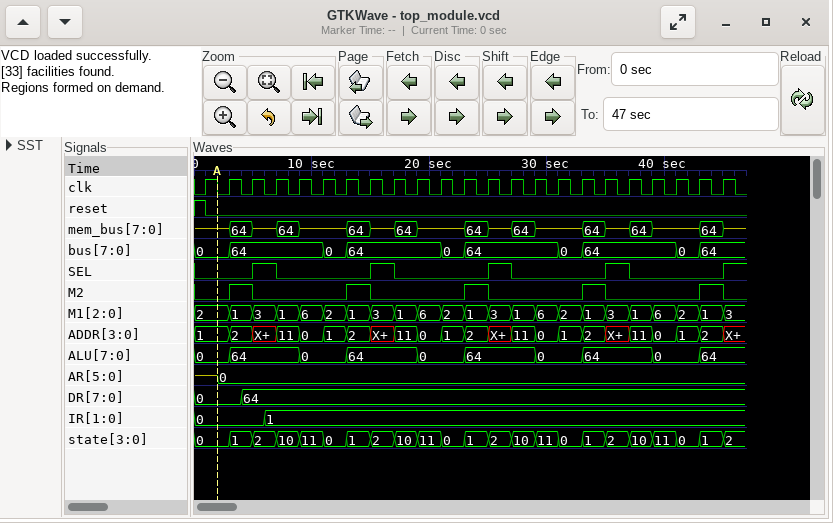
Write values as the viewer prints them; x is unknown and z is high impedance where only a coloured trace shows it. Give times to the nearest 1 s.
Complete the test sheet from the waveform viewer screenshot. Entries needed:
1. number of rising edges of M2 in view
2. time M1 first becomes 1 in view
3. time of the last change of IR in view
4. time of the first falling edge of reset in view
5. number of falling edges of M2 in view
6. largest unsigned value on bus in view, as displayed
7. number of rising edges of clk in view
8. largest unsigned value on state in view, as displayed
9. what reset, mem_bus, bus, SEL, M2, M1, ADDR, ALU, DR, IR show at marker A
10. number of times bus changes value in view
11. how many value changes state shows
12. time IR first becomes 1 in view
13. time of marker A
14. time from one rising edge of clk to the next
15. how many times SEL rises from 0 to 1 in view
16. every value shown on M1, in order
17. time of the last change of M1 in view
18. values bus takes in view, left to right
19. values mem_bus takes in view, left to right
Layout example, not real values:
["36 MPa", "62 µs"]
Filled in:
["5", "3 s", "6 s", "1 s", "5", "64", "23", "11", "reset=0, mem_bus=z, bus=0, SEL=0, M2=0, M1=2, ADDR=1, ALU=0, DR=0, IR=0", "9", "22", "6 s", "2 s", "2 s", "5", "2, 1, 3, 1, 6, 2, 1, 3, 1, 6, 2, 1, 3, 1, 6, 2, 1, 3, 1, 6, 2, 1, 3", "45 s", "0, 64, 0, 64, 0, 64, 0, 64, 0, 64", "z, 64, z, 64, z, 64, z, 64, z, 64, z, 64, z, 64, z, 64, z, 64, z"]
